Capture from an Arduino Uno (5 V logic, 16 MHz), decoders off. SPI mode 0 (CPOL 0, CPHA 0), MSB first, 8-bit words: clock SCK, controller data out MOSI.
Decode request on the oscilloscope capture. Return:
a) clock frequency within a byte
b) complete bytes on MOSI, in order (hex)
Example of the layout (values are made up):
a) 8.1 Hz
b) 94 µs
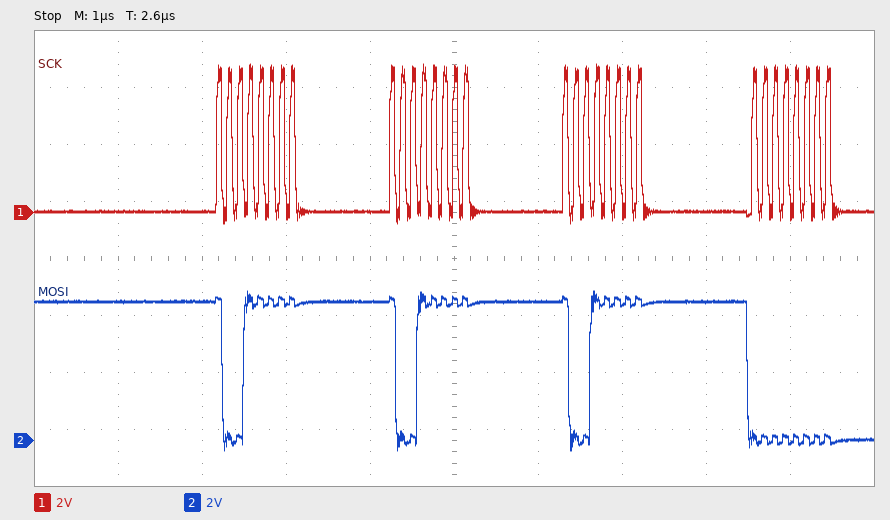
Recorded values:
a) 8 MHz
b) 0x9F 0x9F 0x9F 0x00
